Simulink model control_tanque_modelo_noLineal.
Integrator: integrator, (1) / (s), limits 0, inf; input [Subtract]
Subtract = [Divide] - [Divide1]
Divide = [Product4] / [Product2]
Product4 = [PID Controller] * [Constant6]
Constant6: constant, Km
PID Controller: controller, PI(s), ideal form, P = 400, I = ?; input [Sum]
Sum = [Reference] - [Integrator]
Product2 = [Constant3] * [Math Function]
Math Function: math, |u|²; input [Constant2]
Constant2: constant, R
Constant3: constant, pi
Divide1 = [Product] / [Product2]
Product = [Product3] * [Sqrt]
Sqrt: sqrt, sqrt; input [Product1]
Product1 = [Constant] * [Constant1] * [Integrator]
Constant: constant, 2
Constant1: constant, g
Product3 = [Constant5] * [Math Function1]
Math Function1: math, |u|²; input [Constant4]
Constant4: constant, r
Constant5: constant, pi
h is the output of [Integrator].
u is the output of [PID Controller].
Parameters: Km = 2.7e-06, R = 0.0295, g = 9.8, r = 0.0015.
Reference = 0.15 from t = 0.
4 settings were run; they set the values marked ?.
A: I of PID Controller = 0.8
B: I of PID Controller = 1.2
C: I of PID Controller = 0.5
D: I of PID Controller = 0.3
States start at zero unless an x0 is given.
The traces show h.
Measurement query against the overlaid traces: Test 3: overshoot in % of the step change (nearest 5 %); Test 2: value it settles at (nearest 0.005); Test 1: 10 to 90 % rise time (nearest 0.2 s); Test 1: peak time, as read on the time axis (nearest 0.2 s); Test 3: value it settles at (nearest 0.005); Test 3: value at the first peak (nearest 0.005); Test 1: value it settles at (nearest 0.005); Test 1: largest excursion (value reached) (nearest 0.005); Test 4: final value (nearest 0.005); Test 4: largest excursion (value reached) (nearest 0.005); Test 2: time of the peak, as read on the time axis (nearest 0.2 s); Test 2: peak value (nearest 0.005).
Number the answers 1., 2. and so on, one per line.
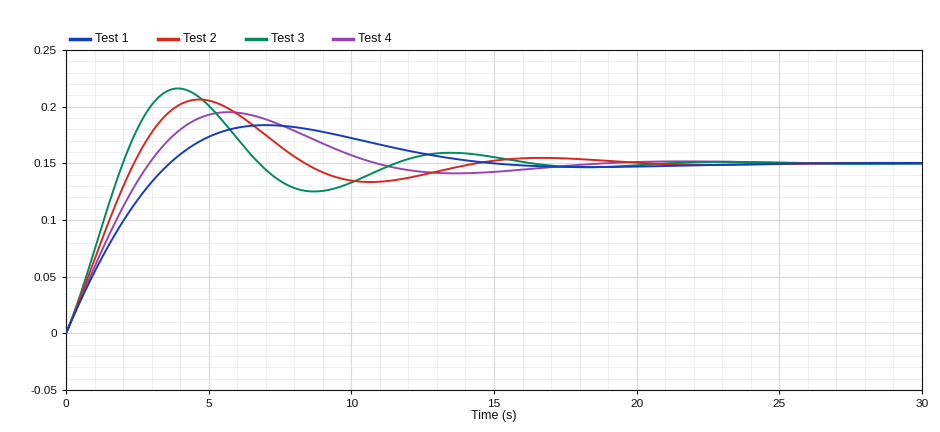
1. 45 %
2. 0.150
3. 2.8 s
4. 7.0 s
5. 0.150
6. 0.215
7. 0.150
8. 0.185
9. 0.150
10. 0.195
11. 4.6 s
12. 0.205
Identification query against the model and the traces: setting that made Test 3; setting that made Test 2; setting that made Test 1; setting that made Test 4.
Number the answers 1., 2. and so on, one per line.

1. B
2. A
3. D
4. C
